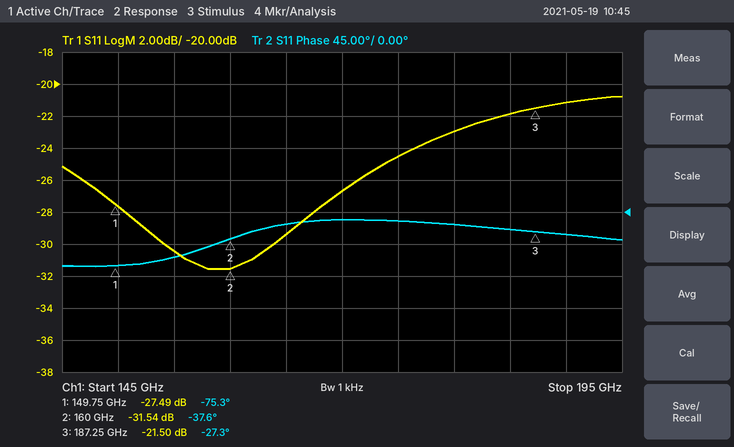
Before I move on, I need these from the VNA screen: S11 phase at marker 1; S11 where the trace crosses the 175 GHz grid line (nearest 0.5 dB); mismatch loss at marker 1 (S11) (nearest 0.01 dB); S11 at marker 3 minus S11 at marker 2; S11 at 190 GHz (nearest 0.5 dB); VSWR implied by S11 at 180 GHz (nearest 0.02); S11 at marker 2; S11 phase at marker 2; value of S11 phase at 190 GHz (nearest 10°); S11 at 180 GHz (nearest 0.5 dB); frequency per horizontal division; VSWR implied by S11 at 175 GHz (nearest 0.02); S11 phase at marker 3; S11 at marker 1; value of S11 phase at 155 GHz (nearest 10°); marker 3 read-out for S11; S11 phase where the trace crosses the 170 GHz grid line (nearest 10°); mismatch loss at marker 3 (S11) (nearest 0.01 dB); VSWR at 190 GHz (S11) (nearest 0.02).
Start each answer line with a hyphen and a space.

- -75.3°
- -24.5 dB
- 0.01 dB
- 10.04 dB
- -21.0 dB
- 1.16
- -31.54 dB
- -37.6°
- -30°
- -23.0 dB
- 5 GHz
- 1.12
- -27.3°
- -27.49 dB
- -60°
- -21.50 dB
- -10°
- 0.03 dB
- 1.20
